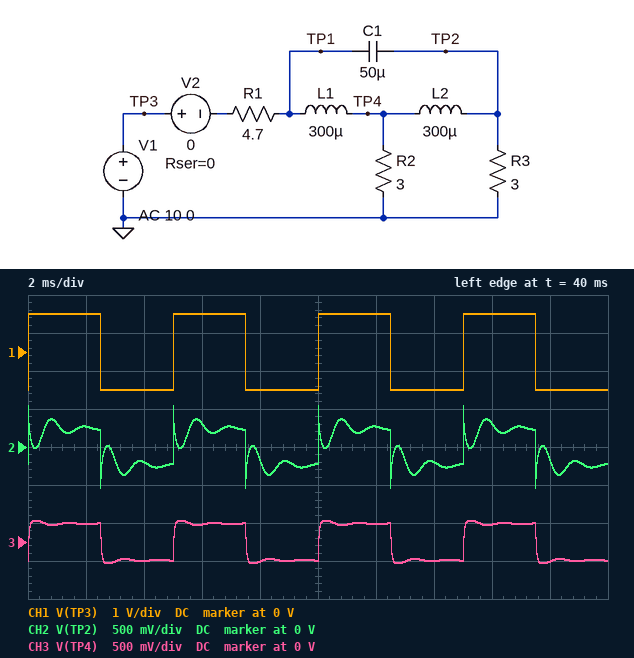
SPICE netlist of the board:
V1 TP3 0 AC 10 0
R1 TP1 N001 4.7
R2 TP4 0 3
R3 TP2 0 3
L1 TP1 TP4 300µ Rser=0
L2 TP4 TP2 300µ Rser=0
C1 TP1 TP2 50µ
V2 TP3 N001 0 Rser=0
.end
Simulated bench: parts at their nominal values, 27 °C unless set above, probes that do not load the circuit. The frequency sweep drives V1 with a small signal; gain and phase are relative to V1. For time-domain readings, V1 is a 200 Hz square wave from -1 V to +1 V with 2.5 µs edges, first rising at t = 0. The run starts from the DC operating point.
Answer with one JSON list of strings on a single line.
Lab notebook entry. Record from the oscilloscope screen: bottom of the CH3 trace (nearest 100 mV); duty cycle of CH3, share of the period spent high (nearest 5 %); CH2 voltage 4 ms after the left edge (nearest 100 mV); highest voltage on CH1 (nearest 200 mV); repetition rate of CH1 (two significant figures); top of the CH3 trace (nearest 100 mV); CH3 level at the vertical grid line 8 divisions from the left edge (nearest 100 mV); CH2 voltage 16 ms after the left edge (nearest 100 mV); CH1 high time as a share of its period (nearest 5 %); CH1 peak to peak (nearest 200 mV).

["-300 mV", "50 %", "-200 mV", "1.0 V", "200 Hz", "300 mV", "200 mV", "300 mV", "50 %", "2.0 V"]
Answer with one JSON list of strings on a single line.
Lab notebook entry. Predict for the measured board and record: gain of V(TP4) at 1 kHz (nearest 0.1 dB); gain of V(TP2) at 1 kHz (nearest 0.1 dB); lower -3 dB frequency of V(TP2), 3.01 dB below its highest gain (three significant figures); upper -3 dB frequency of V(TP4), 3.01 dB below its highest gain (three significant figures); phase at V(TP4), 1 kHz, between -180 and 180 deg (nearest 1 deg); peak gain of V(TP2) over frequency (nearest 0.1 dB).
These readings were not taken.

["-10.7 dB", "-14.6 dB", "1.84 kHz", "2.92 kHz", "-15 deg", "-8.2 dB"]
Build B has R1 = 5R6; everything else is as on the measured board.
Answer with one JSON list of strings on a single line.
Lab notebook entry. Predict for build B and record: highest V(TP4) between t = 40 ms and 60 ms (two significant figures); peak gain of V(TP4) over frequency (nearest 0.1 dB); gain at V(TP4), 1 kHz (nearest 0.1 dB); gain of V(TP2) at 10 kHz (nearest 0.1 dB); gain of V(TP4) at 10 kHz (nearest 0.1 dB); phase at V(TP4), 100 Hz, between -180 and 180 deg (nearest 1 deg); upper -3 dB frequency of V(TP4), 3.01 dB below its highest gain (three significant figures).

["260 mV", "-10.8 dB", "-11.1 dB", "-9.7 dB", "-20.1 dB", "0 deg", "2.00 kHz"]
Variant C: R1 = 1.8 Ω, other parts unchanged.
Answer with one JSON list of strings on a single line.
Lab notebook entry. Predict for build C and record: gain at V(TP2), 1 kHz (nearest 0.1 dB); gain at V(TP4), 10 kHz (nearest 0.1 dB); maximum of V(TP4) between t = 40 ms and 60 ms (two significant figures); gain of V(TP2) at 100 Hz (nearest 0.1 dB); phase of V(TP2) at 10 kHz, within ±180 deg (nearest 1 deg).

["-13.0 dB", "-14.8 dB", "480 mV", "-6.9 dB", "10 deg"]
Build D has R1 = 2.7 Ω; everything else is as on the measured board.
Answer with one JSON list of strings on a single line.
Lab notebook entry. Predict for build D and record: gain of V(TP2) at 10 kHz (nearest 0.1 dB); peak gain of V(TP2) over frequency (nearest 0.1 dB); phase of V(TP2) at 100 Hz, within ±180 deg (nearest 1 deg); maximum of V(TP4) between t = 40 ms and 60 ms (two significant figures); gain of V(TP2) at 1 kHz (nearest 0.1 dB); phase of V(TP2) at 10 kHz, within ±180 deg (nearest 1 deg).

["-6.0 dB", "-5.6 dB", "-5 deg", "360 mV", "-13.5 dB", "11 deg"]
